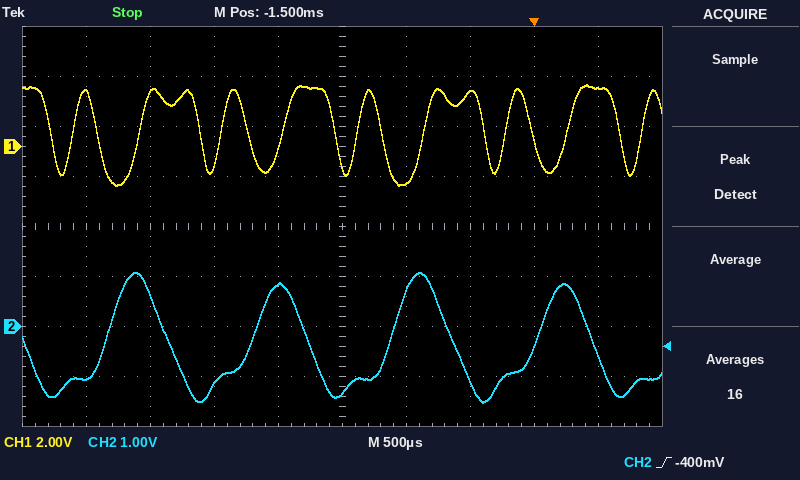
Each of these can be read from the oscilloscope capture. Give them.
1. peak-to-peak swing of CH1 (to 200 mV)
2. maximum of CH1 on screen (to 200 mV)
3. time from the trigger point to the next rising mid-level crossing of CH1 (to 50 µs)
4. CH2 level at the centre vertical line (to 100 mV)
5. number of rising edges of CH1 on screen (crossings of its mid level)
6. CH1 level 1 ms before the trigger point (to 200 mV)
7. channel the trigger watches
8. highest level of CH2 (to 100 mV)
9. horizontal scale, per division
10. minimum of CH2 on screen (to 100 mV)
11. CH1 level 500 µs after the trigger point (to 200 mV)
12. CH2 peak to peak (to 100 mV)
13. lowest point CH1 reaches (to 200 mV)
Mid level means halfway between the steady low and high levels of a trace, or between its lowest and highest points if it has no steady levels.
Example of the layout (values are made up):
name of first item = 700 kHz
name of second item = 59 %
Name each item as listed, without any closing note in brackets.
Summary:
peak-to-peak swing of CH1 = 4.0 V
maximum of CH1 on screen = 2.4 V
time from the trigger point to the next rising mid-level crossing of CH1 = 250 µs
CH2 level at the centre vertical line = -1.3 V
number of rising edges of CH1 on screen = 9
CH1 level 1 ms before the trigger point = -1.4 V
channel the trigger watches = CH2
highest level of CH2 = 1.1 V
horizontal scale, per division = 500 µs
minimum of CH2 on screen = -1.5 V
CH1 level 500 µs after the trigger point = 2.4 V
CH2 peak to peak = 2.6 V
lowest point CH1 reaches = -1.6 V
